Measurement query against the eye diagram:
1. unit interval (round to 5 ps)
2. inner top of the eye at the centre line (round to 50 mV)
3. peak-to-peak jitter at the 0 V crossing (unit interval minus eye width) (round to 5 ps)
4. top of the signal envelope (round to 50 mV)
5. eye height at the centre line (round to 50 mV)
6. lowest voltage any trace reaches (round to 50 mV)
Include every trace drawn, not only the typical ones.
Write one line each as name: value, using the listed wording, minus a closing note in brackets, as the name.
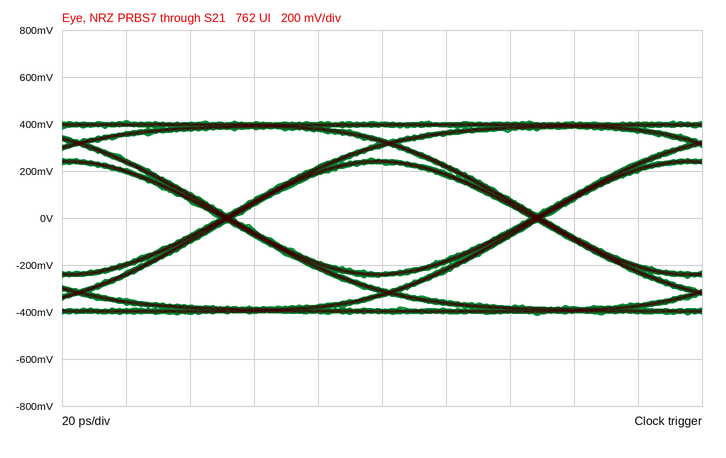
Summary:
unit interval: 95 ps
inner top of the eye at the centre line: 250 mV
peak-to-peak jitter at the 0 V crossing (unit interval minus eye width): 5 ps
top of the signal envelope: 400 mV
eye height at the centre line: 450 mV
lowest voltage any trace reaches: -400 mV
